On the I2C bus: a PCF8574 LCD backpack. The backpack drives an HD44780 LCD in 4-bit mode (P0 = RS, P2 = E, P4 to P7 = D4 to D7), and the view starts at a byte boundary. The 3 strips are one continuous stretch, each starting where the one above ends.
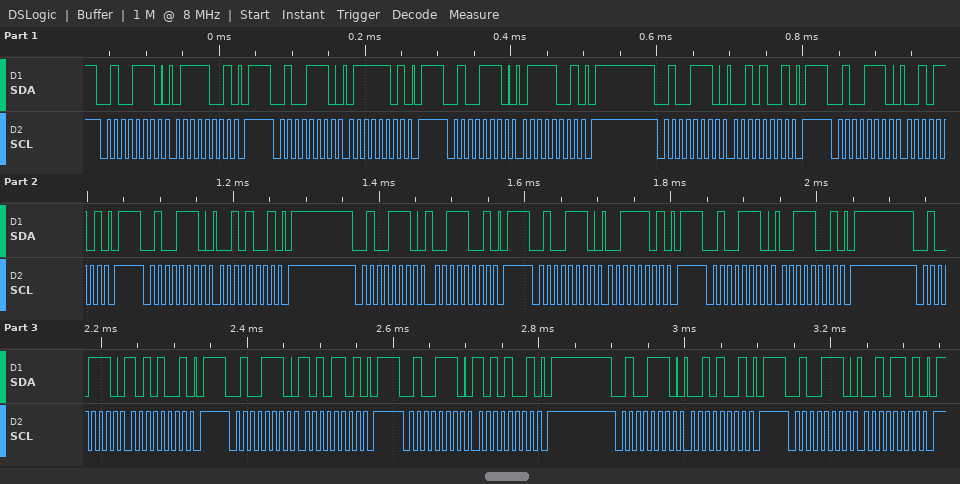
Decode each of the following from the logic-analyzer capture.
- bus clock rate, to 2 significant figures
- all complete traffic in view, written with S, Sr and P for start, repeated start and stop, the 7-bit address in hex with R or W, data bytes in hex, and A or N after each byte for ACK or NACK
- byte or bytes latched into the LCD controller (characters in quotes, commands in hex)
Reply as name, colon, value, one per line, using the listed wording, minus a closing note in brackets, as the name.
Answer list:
bus clock rate, to 2 significant figures: 100 kHz
all complete traffic in view, written with S, Sr and P for start, repeated start and stop, the 7-bit address in hex with R or W, data bytes in hex, and A or N after each byte for ACK or NACK: S 27W A 79 A P S 27W A 7D A P S 27W A 79 A P S 27W A 29 A P S 27W A 2D A P S 27W A 29 A P S 27W A 39 A P S 27W A 3D A P S 27W A 39 A P S 27W A A9 A P S 27W A AD A P S 27W A A9 A P S 27W A 29 A P S 27W A 2D A P
byte or bytes latched into the LCD controller: 'r' ':'
